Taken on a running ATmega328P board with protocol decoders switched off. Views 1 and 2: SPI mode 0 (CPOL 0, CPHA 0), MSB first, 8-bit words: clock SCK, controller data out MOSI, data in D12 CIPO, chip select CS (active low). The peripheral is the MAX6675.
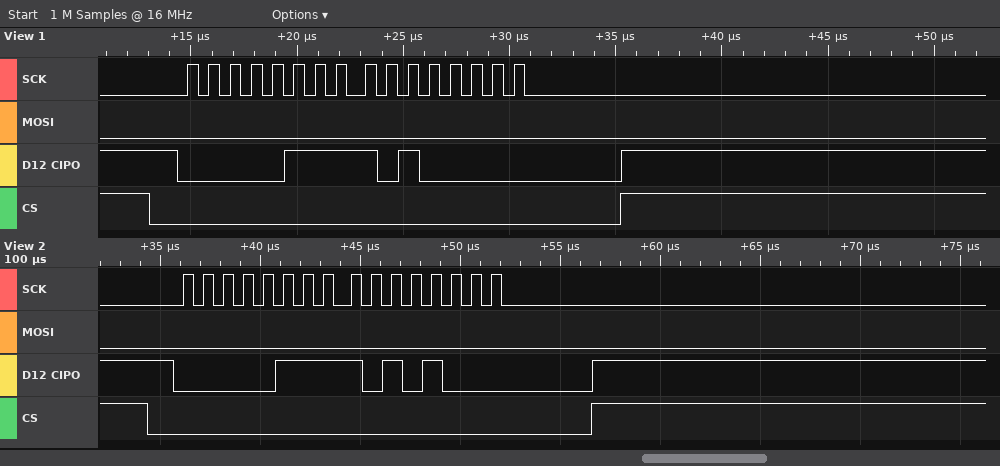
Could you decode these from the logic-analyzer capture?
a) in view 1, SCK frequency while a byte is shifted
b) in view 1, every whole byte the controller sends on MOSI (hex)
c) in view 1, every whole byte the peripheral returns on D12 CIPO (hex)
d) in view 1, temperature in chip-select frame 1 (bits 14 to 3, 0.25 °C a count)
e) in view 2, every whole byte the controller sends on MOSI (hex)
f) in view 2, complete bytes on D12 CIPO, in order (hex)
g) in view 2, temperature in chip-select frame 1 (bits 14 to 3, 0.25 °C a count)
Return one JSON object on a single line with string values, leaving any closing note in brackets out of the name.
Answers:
{"in view 1, SCK frequency while a byte is shifted": "1 MHz", "in view 1, every whole byte the controller sends on MOSI": "00 00", "in view 1, every whole byte the peripheral returns on D12 CIPO": "07 A0", "in view 1, temperature in chip-select frame 1": "61.00 °C", "in view 2, every whole byte the controller sends on MOSI": "00 00", "in view 2, complete bytes on D12 CIPO, in order": "07 A8", "in view 2, temperature in chip-select frame 1": "61.25 °C"}
